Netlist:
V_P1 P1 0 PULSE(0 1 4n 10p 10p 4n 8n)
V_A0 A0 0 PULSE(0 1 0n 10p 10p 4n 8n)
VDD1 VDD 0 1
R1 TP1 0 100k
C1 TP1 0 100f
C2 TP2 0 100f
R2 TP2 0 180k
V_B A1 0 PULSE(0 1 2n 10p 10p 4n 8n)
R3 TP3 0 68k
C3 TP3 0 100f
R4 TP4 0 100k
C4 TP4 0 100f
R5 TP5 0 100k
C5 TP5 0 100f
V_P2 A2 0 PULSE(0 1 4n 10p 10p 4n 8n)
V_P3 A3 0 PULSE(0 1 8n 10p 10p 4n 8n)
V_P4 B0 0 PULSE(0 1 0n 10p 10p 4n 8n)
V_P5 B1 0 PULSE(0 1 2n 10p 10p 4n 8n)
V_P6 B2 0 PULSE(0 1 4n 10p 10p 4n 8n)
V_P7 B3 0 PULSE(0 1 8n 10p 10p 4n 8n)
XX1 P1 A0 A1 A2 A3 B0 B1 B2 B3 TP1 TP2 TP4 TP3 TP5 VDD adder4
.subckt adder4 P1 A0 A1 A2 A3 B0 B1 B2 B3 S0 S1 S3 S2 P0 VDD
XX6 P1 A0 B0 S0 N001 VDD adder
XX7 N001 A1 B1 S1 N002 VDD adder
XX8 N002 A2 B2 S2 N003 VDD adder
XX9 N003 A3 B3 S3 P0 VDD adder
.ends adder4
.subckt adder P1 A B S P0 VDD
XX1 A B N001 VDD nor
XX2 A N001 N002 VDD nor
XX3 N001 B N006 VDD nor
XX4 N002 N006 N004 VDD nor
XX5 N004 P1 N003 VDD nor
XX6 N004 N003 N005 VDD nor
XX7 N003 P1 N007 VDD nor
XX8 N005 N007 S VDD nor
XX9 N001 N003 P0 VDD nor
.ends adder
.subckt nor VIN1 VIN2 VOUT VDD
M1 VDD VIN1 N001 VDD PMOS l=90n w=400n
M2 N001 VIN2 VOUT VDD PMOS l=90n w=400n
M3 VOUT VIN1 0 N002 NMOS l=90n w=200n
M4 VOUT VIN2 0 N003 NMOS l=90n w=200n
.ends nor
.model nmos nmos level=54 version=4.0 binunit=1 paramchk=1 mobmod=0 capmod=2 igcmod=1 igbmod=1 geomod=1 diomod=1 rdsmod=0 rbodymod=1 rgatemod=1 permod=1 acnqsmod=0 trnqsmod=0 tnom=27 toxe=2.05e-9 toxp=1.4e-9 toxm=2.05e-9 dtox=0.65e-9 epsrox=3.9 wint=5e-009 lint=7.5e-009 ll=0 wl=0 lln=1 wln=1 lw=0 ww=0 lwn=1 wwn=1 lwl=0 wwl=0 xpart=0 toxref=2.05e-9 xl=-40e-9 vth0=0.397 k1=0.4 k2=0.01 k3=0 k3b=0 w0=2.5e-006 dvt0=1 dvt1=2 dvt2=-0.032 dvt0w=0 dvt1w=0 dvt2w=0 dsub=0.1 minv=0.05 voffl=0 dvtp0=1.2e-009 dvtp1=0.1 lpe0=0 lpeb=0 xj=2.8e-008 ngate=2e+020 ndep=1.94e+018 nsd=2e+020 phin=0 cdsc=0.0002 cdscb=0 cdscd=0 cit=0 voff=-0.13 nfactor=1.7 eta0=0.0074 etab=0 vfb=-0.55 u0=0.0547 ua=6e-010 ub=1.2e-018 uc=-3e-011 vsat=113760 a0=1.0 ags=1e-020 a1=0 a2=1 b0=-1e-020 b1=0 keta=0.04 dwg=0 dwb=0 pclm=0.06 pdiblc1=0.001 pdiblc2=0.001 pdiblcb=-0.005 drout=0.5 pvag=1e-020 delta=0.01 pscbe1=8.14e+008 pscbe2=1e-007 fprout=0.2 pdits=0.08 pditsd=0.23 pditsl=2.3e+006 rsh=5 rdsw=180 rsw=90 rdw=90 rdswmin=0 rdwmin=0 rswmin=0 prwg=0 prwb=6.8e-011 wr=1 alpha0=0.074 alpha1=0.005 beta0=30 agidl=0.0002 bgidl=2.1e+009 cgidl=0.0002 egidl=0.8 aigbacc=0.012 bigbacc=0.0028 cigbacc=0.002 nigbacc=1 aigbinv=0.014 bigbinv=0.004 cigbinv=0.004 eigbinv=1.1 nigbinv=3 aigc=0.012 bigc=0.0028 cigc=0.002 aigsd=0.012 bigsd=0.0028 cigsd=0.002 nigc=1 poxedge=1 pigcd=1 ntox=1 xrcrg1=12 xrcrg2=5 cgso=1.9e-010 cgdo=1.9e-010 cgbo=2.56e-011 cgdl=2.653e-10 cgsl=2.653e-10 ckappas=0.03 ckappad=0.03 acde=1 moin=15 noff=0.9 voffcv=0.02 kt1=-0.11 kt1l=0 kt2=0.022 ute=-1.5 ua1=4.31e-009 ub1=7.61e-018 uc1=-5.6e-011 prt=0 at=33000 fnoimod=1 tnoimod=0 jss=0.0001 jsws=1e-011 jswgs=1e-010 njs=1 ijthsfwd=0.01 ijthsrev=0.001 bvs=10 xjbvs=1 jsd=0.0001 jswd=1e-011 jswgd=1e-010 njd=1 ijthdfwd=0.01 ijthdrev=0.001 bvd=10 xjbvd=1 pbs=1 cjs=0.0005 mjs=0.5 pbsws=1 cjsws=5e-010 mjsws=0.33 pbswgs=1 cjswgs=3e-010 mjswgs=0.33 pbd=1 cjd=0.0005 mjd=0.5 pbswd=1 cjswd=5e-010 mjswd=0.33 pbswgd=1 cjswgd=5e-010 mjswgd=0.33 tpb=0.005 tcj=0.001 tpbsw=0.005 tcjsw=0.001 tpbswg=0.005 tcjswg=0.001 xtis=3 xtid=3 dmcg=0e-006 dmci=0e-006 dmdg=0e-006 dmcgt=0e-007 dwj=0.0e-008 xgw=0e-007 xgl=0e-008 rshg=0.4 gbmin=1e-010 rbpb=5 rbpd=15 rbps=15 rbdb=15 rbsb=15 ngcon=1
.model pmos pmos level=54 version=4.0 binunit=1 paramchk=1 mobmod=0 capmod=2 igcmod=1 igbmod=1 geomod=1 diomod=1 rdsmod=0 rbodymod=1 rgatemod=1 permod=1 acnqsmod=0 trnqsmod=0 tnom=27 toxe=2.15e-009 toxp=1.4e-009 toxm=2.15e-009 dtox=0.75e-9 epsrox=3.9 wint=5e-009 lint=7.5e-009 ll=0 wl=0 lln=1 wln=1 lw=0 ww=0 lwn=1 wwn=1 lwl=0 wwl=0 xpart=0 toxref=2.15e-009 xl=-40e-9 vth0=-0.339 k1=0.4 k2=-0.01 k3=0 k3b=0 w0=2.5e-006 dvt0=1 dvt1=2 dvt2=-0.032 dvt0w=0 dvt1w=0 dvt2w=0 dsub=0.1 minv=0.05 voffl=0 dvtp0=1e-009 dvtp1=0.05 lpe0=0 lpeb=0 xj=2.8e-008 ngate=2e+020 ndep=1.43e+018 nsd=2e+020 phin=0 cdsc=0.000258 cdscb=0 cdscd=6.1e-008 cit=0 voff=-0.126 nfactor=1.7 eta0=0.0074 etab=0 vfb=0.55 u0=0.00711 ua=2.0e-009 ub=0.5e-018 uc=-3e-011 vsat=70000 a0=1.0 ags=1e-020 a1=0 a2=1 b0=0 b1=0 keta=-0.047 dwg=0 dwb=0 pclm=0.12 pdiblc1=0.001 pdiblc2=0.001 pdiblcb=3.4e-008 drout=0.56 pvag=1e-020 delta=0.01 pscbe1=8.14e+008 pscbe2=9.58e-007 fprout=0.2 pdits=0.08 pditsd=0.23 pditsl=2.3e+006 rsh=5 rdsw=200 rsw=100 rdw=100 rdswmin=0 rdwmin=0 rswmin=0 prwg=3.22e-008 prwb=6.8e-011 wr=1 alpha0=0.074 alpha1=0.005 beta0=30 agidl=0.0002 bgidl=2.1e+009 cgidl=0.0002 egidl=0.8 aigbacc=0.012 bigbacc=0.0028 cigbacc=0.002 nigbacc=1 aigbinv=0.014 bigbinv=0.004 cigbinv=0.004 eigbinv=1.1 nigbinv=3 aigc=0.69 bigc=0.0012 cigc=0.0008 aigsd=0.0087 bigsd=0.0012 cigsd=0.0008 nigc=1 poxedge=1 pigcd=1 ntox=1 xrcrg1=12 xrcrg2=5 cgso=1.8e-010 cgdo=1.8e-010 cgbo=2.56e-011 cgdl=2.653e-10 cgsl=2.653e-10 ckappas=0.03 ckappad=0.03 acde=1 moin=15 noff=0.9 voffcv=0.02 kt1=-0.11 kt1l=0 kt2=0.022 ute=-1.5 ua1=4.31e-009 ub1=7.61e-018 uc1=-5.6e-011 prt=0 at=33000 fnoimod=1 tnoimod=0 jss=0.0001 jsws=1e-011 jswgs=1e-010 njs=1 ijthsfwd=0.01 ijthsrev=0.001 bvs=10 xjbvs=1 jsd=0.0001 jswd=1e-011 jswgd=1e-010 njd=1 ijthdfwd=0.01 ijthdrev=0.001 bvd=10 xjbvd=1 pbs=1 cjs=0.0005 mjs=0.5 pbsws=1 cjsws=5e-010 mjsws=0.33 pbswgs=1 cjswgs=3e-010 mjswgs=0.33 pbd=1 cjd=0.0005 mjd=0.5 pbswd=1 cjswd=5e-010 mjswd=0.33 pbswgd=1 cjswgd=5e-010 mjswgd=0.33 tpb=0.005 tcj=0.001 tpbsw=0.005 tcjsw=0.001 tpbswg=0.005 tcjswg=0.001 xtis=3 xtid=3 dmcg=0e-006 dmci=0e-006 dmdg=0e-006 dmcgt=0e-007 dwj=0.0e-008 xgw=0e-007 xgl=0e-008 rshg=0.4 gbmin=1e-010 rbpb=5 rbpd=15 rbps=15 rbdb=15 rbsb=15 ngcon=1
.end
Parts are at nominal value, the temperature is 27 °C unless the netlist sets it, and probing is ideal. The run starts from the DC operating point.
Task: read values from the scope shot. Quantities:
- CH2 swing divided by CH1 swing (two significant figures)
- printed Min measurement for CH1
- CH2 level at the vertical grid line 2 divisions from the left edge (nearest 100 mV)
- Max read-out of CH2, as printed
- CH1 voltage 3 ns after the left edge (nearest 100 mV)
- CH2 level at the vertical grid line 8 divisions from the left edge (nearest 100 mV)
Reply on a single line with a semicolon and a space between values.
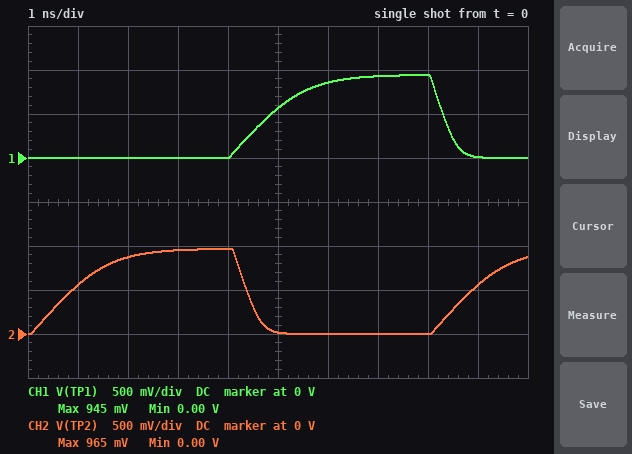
1.0; 0.00 V; 900 mV; 965 mV; 0 V; 0 V
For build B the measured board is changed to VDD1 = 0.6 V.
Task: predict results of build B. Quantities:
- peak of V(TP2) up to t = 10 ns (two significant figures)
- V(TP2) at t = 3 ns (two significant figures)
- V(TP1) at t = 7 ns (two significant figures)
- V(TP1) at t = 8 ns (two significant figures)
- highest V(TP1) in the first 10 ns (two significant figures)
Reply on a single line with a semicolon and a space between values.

470 mV; 370 mV; 360 mV; 430 mV; 440 mV
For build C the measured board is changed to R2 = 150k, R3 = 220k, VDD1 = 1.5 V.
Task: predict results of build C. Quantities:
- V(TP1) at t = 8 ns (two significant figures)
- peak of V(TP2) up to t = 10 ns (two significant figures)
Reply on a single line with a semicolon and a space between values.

1.4 V; 1.5 V
